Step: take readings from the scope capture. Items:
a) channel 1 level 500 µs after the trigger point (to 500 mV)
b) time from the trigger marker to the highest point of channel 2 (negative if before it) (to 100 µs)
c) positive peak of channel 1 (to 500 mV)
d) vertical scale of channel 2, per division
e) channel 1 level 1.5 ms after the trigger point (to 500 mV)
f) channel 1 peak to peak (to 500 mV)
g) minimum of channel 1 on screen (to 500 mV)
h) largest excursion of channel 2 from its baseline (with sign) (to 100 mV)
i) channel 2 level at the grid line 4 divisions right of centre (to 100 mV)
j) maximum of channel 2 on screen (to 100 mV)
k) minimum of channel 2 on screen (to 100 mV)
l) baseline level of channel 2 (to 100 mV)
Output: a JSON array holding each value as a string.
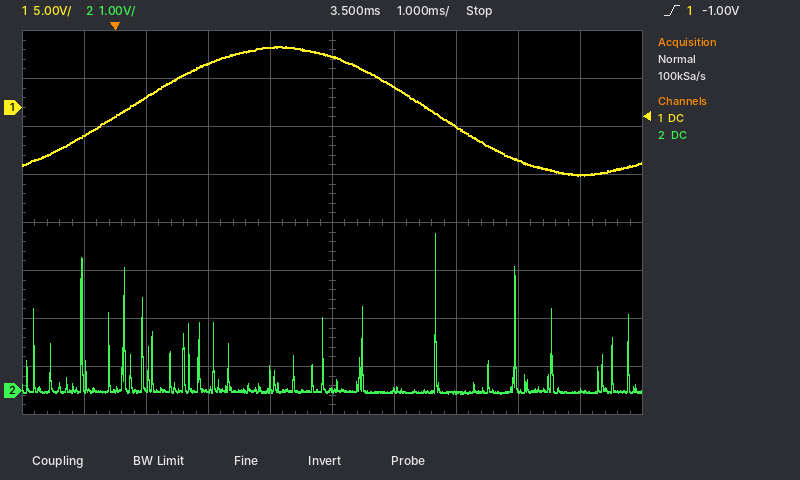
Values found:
["1.0 V", "+5.2 ms", "6.5 V", "1 V", "4.5 V", "13.5 V", "-7.0 V", "+3.3 V", "0.0 V", "3.3 V", "-100 mV", "0.0 V"]
